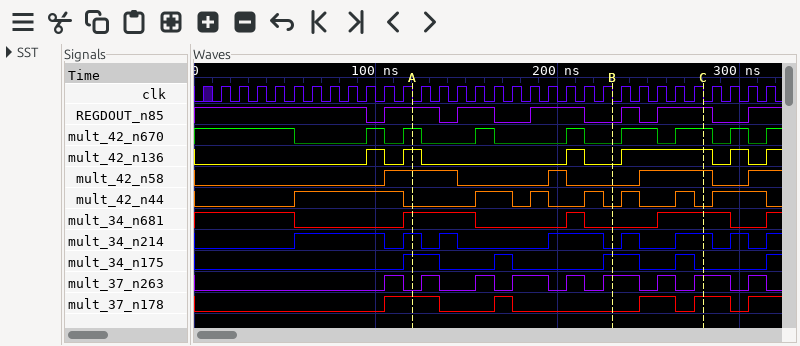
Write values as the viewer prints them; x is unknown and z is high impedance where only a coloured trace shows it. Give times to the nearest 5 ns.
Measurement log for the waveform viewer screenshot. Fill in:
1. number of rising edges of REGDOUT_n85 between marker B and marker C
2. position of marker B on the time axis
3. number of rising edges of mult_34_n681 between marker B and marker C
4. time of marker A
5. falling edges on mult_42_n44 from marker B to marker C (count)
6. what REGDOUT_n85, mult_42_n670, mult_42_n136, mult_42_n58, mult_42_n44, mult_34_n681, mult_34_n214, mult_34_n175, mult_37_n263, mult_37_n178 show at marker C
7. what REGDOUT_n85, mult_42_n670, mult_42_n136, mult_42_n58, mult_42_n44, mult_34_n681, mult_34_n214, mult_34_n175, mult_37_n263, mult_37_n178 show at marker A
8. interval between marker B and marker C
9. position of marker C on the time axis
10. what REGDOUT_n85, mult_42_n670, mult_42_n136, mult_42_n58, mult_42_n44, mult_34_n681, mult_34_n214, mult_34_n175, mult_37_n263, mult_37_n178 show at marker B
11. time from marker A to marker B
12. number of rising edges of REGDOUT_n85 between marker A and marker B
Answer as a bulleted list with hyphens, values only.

- 2
- 230 ns
- 1
- 120 ns
- 2
- REGDOUT_n85=1, mult_42_n670=1, mult_42_n136=1, mult_42_n58=1, mult_42_n44=0, mult_34_n681=1, mult_34_n214=1, mult_34_n175=0, mult_37_n263=1, mult_37_n178=1
- REGDOUT_n85=1, mult_42_n670=1, mult_42_n136=1, mult_42_n58=1, mult_42_n44=0, mult_34_n681=1, mult_34_n214=1, mult_34_n175=1, mult_37_n263=0, mult_37_n178=1
- 50 ns
- 280 ns
- REGDOUT_n85=0, mult_42_n670=0, mult_42_n136=0, mult_42_n58=0, mult_42_n44=0, mult_34_n681=0, mult_34_n214=0, mult_34_n175=1, mult_37_n263=1, mult_37_n178=0
- 110 ns
- 2
